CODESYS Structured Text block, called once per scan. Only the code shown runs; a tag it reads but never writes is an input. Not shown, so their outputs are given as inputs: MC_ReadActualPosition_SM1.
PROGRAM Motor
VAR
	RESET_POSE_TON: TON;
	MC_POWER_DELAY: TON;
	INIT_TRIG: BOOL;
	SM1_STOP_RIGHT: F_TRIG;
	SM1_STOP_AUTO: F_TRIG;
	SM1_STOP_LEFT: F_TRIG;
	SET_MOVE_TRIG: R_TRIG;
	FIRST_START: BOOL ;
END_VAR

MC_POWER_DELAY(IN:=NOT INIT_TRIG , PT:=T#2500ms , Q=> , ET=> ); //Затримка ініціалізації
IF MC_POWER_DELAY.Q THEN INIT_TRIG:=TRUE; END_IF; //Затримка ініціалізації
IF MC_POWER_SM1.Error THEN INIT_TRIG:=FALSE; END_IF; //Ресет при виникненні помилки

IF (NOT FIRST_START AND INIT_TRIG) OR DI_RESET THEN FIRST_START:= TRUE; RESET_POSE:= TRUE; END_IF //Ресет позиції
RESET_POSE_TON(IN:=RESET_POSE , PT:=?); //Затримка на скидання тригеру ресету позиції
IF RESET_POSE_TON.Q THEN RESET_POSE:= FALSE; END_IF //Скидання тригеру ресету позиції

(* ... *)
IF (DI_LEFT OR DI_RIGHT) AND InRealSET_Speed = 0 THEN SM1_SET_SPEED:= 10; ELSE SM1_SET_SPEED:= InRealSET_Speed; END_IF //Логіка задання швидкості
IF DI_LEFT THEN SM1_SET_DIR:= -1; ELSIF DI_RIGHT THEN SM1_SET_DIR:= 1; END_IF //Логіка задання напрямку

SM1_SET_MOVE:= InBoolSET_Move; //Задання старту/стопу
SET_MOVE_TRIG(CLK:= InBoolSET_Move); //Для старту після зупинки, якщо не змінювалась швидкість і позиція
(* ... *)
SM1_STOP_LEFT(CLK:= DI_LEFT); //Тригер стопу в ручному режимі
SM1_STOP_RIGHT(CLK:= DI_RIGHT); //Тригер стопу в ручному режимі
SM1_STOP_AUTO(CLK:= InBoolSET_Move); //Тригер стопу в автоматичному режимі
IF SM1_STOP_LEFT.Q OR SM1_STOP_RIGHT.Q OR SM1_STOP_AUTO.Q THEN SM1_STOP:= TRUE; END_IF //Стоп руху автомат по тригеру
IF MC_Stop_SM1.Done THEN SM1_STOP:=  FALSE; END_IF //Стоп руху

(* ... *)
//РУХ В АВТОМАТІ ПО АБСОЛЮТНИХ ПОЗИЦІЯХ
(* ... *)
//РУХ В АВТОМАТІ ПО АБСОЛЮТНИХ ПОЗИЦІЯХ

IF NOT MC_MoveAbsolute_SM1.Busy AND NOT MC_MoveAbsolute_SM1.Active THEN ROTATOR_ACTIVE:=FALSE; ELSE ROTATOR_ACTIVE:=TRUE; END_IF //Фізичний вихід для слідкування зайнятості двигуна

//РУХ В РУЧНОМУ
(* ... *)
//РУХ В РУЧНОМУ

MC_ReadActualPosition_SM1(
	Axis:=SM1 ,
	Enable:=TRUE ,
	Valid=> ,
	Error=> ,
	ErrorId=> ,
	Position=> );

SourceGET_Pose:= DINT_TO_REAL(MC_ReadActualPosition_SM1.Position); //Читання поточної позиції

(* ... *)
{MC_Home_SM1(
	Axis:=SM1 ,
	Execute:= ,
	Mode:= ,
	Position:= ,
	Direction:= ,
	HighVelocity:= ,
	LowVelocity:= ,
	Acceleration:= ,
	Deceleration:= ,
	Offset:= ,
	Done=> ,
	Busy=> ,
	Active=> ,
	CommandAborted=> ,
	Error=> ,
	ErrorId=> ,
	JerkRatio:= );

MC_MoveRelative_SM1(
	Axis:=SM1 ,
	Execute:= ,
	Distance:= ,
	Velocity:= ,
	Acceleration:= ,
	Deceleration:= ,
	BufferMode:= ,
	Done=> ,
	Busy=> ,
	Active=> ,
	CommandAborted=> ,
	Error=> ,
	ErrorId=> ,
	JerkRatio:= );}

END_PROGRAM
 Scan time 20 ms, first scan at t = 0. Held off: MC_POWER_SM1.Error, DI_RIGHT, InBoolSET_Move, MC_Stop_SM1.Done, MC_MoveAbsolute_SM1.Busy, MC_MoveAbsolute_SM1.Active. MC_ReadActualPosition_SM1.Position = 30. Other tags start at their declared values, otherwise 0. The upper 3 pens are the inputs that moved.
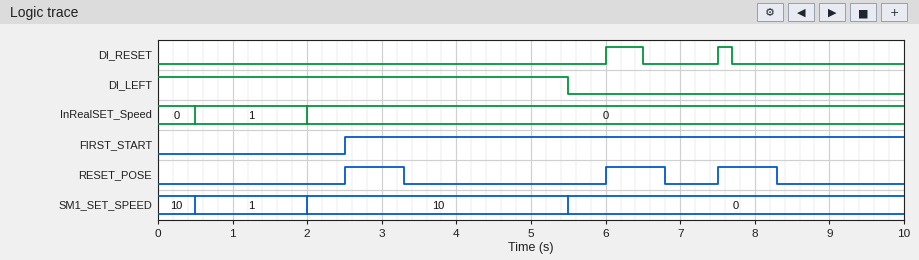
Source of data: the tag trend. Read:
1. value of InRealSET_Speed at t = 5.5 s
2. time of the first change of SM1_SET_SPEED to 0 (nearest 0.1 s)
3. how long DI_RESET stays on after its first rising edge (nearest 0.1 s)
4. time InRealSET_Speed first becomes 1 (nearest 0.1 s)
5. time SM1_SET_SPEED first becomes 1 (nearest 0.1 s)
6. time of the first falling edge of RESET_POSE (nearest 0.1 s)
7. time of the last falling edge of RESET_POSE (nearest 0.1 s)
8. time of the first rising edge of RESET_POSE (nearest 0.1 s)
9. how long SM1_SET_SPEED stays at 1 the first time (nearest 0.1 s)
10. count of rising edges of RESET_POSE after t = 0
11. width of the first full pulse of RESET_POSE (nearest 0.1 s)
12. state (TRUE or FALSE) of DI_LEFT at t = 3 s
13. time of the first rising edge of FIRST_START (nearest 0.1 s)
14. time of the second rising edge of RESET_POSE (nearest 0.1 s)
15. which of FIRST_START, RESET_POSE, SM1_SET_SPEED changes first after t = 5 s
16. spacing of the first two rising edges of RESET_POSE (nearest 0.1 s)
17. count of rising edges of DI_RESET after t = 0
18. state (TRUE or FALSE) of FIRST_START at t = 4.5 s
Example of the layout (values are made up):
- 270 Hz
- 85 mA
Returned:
- 0
- 5.5 s
- 0.5 s
- 0.5 s
- 0.5 s
- 3.3 s
- 8.3 s
- 2.5 s
- 1.5 s
- 3
- 0.8 s
- TRUE
- 2.5 s
- 6.0 s
- SM1_SET_SPEED
- 3.5 s
- 2
- TRUE
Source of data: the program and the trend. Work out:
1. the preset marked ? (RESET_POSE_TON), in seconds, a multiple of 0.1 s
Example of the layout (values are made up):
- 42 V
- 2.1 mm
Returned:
- 0.8 s
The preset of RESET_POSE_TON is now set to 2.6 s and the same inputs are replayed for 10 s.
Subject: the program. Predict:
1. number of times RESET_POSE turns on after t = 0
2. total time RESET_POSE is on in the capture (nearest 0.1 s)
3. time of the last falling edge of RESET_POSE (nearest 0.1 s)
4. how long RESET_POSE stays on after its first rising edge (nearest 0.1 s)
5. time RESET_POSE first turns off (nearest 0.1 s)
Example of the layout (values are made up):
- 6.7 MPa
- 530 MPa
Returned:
- 2
- 5.2 s
- 8.6 s
- 2.6 s
- 5.1 s
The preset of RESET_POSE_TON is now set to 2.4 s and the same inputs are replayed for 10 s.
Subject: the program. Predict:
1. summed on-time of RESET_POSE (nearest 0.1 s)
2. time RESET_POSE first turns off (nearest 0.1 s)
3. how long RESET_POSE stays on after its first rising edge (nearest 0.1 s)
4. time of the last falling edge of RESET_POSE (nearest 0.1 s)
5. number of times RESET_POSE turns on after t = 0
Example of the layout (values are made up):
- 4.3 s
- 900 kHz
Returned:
- 4.8 s
- 4.9 s
- 2.4 s
- 8.4 s
- 2
